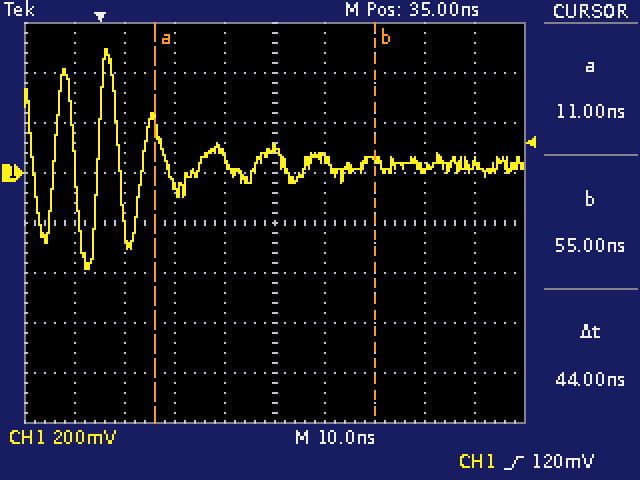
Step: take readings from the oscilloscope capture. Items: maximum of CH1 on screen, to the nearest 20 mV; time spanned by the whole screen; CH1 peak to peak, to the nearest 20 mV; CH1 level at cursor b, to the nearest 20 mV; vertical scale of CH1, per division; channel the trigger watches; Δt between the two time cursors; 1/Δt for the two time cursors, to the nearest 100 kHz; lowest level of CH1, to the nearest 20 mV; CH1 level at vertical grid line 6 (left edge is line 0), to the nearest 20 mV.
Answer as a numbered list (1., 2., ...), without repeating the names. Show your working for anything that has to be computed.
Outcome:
1. 500 mV
2. 100 ns
3. 500 mV − (-380 mV) = 880 mV
4. 40 mV
5. 200 mV
6. CH1
7. 44 ns
8. 1 / 44 ns ≈ 22.7 MHz
9. -380 mV
10. 60 mV
